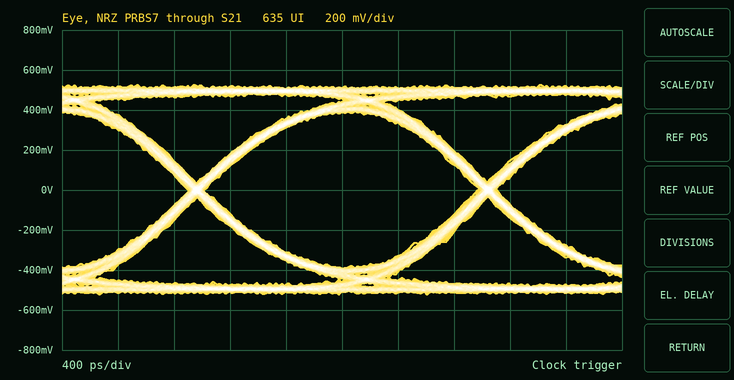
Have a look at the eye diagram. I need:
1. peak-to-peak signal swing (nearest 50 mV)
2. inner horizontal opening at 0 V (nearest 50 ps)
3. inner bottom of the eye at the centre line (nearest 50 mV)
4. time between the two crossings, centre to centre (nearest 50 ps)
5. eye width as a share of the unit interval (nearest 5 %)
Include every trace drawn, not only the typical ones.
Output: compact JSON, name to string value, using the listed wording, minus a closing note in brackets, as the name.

{"peak-to-peak signal swing": "1.05 V", "inner horizontal opening at 0 V": "1.95 ns", "inner bottom of the eye at the centre line": "-400 mV", "time between the two crossings, centre to centre": "2.10 ns", "eye width as a share of the unit interval": "95 %"}
